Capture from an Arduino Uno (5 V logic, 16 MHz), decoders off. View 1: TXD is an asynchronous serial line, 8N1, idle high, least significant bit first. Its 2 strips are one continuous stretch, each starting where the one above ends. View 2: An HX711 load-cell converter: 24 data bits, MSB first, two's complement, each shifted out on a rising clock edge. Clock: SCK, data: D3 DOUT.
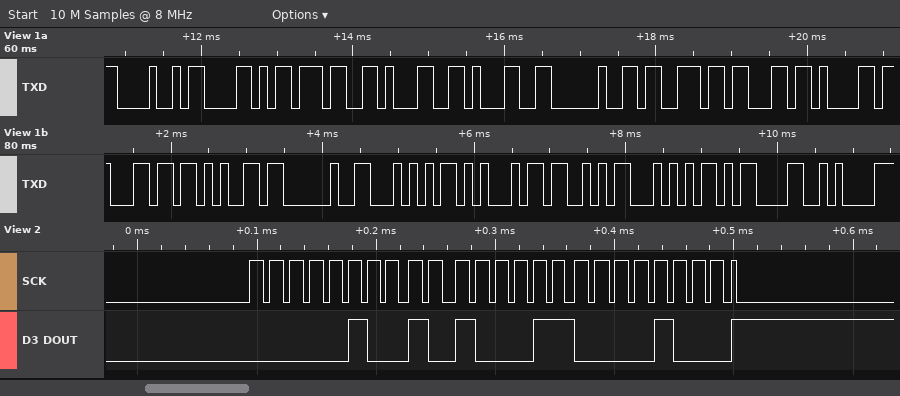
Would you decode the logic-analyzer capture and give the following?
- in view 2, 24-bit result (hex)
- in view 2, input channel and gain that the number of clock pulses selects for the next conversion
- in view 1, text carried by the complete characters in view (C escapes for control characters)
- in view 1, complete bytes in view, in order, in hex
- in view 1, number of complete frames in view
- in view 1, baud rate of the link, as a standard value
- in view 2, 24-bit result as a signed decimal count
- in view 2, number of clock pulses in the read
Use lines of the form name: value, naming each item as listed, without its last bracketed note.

in view 2, 24-bit result: 0x04A308
in view 2, input channel and gain that the number of clock pulses selects for the next conversion: channel A, gain 128
in view 1, text carried by the complete characters in view: "HX711 scale TEST\r\n"
in view 1, complete bytes in view, in order, in hex: 0x48 0x58 0x37 0x31 0x31 0x20 0x73 0x63 0x61 0x6C 0x65 0x20 0x54 0x45 0x53 0x54 0x0D 0x0A
in view 1, number of complete frames in view: 18
in view 1, baud rate of the link, as a standard value: 9600 baud
in view 2, 24-bit result as a signed decimal count: 303880
in view 2, number of clock pulses in the read: 25
